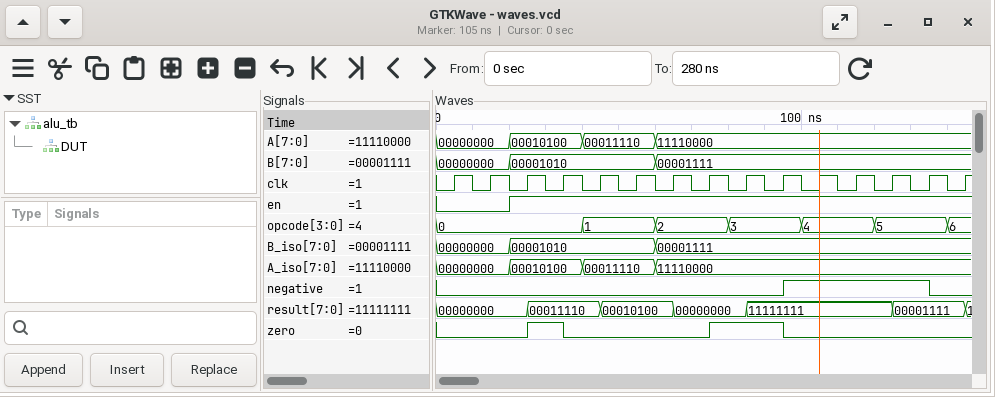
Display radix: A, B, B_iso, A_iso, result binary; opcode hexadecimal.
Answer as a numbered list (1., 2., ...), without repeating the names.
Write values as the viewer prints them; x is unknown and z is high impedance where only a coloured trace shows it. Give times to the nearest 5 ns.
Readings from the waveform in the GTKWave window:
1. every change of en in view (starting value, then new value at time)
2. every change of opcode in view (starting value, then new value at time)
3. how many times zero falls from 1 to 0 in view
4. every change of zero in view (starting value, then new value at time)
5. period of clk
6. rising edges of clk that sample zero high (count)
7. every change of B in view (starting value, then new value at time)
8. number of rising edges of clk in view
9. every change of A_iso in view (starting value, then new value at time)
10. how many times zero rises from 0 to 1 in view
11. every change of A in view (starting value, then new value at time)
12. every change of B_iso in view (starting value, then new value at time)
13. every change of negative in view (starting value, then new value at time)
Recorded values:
1. 0, 1 at 20 ns
2. 0, 1 at 40 ns, 2 at 60 ns, 3 at 80 ns, 4 at 100 ns, 5 at 120 ns, 6 at 140 ns
3. 2
4. 0, 1 at 25 ns, 0 at 35 ns, 1 at 75 ns, 0 at 95 ns
5. 10 ns
6. 3
7. 00000000, 00001010 at 20 ns, 00001111 at 60 ns
8. 15
9. 00000000, 00010100 at 20 ns, 00011110 at 40 ns, 11110000 at 60 ns
10. 2
11. 00000000, 00010100 at 20 ns, 00011110 at 40 ns, 11110000 at 60 ns
12. 00000000, 00001010 at 20 ns, 00001111 at 60 ns
13. 0, 1 at 95 ns, 0 at 135 ns
